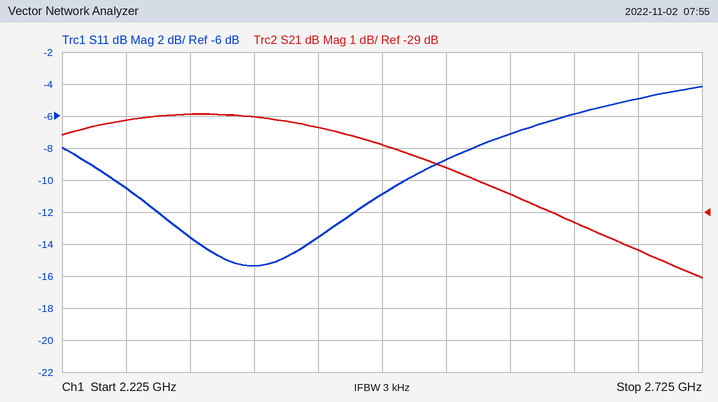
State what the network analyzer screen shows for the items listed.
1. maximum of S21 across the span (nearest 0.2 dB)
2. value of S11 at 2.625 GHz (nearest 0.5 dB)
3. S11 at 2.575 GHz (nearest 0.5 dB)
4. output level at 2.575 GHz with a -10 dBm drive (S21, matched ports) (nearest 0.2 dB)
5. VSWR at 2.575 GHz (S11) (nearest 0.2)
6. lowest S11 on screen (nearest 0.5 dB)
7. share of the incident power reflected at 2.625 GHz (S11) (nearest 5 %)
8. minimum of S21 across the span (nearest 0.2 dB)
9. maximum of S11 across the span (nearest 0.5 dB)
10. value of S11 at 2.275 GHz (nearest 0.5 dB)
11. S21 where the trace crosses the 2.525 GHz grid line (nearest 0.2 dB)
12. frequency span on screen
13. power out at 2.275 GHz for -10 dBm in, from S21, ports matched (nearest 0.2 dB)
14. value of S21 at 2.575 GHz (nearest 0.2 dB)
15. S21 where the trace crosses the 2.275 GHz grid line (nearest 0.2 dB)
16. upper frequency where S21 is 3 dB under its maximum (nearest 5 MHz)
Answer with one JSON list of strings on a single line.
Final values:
["-26.0 dB", "-6.0 dB", "-7.0 dB", "-38.4 dBm", "2.6", "-15.5 dB", "25 %", "-31.0 dB", "-4.0 dB", "-10.5 dB", "-27.6 dB", "500 MHz", "-36.2 dBm", "-28.4 dB", "-26.2 dB", "2.605 GHz"]
